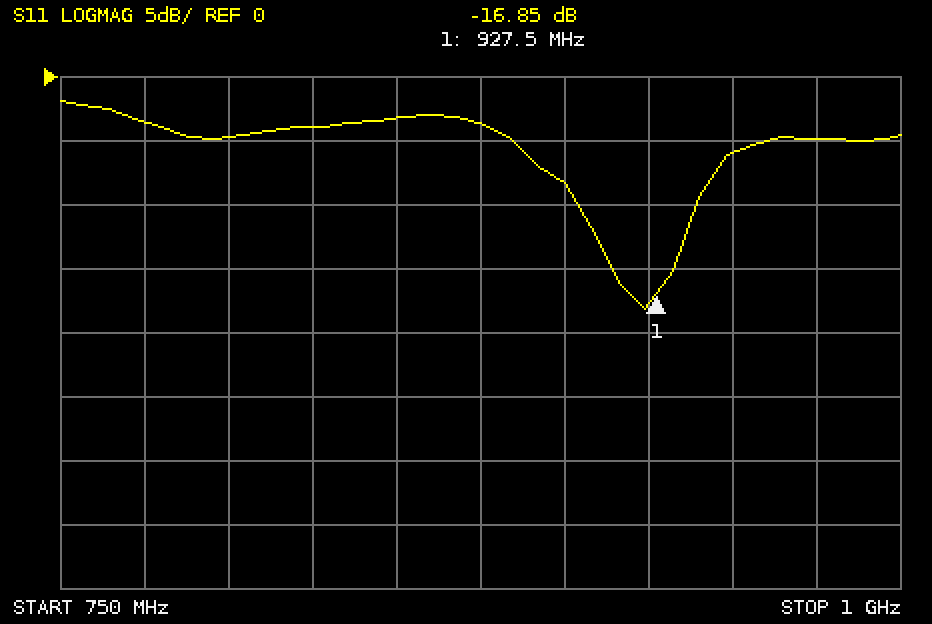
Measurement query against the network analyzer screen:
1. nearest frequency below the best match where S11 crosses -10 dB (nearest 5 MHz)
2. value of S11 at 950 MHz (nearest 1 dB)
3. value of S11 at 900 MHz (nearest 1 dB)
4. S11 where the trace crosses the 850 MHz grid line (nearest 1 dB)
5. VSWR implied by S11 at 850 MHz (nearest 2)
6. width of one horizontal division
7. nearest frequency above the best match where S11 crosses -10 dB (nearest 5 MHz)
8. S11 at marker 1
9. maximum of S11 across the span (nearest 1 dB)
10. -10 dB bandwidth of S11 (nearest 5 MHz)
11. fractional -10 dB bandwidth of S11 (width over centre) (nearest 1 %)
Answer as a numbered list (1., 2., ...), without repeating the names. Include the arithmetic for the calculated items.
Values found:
1. 905 MHz
2. -6 dB
3. -8 dB
4. -3 dB
5. |Γ| = 10^(-3/20) = 0.7079; VSWR = (1 + 0.7079)/(1 − 0.7079) ≈ 6
6. 25 MHz
7. 940 MHz
8. -16.85 dB
9. -2 dB
10. 940 MHz − 905 MHz = 35 MHz
11. 35 MHz / 922.5 MHz ≈ 4 %
